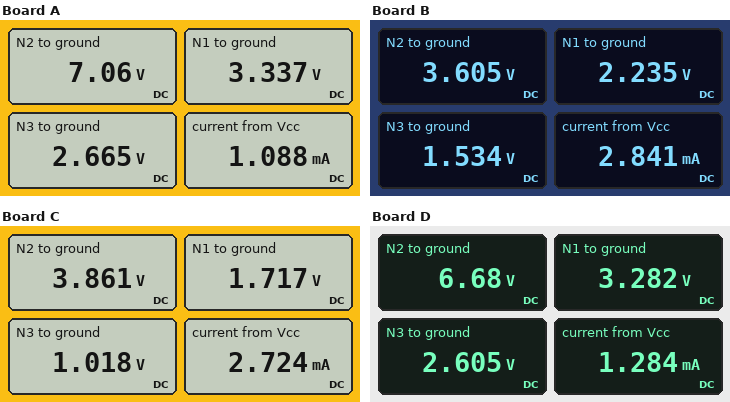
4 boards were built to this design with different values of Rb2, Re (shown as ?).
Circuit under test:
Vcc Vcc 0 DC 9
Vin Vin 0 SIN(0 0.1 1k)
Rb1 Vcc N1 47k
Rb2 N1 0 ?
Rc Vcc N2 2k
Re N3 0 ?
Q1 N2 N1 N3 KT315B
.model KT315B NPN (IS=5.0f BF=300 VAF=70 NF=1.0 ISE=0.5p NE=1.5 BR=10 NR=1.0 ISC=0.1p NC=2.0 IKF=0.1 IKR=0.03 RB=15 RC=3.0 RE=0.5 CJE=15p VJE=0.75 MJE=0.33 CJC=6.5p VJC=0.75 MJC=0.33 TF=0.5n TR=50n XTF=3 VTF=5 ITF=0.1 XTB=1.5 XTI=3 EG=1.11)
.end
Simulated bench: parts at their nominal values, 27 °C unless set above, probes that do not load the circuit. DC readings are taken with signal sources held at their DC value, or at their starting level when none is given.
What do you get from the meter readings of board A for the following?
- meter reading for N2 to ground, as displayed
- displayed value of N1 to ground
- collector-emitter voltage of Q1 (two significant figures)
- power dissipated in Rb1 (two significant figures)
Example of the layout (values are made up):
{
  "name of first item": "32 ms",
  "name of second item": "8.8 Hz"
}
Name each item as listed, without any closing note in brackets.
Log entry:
{
  "meter reading for N2 to ground, as displayed": "7.06 V",
  "displayed value of N1 to ground": "3.337 V",
  "collector-emitter voltage of Q1": "4.4 V",
  "power dissipated in Rb1": "680 µW"
}
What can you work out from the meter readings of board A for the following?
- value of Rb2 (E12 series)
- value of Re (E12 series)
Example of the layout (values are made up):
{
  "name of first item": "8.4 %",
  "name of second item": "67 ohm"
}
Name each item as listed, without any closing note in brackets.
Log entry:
{
  "value of Rb2": "33 kΩ",
  "value of Re": "2.7 kΩ"
}
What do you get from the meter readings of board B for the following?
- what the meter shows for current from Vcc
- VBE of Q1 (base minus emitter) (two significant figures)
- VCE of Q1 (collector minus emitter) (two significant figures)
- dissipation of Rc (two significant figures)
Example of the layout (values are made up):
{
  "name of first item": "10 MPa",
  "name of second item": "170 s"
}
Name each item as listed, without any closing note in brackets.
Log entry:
{
  "what the meter shows for current from Vcc": "2.841 mA",
  "VBE of Q1 (base minus emitter)": "700 mV",
  "VCE of Q1 (collector minus emitter)": "2.1 V",
  "dissipation of Rc": "15 mW"
}
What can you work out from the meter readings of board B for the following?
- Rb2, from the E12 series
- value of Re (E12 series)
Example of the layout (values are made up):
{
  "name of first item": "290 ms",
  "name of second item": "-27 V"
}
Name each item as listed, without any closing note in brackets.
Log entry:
{
  "Rb2, from the E12 series": "22 kΩ",
  "value of Re": "560 Ω"
}
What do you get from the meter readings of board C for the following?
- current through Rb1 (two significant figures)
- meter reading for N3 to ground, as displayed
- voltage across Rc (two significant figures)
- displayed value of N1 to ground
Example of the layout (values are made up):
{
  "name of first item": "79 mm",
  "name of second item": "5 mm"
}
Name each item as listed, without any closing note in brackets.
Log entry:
{
  "current through Rb1": "150 µA",
  "meter reading for N3 to ground, as displayed": "1.018 V",
  "voltage across Rc": "5.1 V",
  "displayed value of N1 to ground": "1.717 V"
}
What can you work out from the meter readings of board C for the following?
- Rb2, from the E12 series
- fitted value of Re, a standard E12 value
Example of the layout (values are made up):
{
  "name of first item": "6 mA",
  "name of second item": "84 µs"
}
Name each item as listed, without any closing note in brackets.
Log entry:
{
  "Rb2, from the E12 series": "15 kΩ",
  "fitted value of Re, a standard E12 value": "390 Ω"
}
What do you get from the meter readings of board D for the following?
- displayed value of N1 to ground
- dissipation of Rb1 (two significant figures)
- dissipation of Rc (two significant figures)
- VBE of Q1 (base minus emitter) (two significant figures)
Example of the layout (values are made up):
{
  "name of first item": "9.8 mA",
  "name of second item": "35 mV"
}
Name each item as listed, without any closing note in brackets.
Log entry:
{
  "displayed value of N1 to ground": "3.282 V",
  "dissipation of Rb1": "700 µW",
  "dissipation of Rc": "2.7 mW",
  "VBE of Q1 (base minus emitter)": "680 mV"
}
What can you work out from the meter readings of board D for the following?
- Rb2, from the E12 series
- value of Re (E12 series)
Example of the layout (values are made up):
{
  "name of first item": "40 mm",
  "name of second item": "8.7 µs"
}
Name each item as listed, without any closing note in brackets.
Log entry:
{
  "Rb2, from the E12 series": "33 kΩ",
  "value of Re": "2.2 kΩ"
}
